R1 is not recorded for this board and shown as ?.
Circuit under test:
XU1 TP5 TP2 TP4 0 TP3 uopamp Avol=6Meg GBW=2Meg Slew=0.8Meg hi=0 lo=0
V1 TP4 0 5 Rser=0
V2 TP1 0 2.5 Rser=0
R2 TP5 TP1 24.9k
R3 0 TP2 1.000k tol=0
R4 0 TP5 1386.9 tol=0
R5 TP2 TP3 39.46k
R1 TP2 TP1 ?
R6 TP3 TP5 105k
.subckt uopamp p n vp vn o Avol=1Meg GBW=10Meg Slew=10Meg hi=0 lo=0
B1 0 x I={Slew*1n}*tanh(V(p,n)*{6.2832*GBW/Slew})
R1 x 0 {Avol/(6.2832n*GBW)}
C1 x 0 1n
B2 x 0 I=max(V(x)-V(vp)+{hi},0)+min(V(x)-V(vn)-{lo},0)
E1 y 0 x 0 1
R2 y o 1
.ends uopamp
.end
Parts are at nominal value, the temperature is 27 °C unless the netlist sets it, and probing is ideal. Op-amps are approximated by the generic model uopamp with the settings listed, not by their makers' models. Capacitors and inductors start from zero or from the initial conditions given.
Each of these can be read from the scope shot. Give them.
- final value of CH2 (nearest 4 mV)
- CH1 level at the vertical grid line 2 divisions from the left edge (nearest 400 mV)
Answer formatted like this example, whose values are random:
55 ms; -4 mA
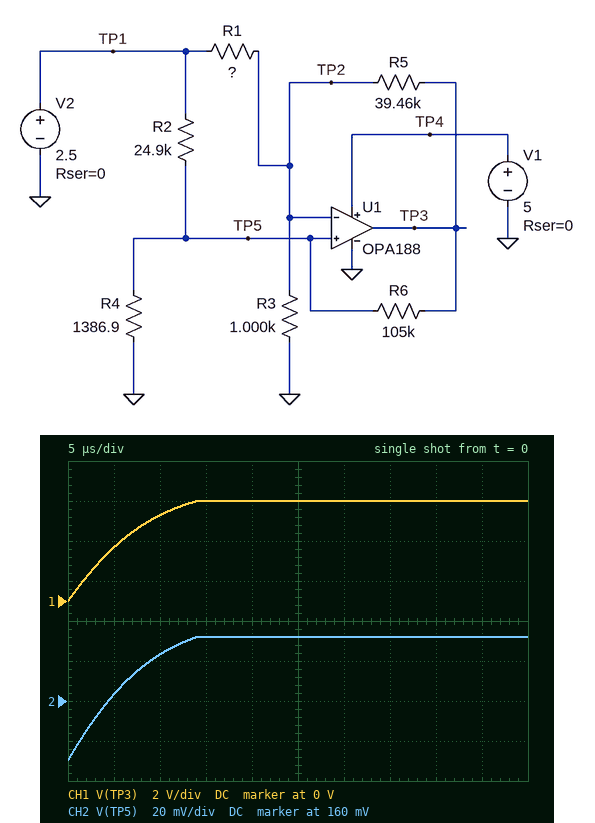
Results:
192 mV; 4.4 V
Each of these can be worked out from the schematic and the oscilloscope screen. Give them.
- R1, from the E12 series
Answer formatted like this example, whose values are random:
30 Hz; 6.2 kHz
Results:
39 kΩ
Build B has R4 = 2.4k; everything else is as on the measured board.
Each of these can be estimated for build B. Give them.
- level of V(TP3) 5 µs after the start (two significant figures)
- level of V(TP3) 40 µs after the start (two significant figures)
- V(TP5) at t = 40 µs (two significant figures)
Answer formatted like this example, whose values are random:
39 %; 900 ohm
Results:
3.9 V; 5.0 V; 320 mV
